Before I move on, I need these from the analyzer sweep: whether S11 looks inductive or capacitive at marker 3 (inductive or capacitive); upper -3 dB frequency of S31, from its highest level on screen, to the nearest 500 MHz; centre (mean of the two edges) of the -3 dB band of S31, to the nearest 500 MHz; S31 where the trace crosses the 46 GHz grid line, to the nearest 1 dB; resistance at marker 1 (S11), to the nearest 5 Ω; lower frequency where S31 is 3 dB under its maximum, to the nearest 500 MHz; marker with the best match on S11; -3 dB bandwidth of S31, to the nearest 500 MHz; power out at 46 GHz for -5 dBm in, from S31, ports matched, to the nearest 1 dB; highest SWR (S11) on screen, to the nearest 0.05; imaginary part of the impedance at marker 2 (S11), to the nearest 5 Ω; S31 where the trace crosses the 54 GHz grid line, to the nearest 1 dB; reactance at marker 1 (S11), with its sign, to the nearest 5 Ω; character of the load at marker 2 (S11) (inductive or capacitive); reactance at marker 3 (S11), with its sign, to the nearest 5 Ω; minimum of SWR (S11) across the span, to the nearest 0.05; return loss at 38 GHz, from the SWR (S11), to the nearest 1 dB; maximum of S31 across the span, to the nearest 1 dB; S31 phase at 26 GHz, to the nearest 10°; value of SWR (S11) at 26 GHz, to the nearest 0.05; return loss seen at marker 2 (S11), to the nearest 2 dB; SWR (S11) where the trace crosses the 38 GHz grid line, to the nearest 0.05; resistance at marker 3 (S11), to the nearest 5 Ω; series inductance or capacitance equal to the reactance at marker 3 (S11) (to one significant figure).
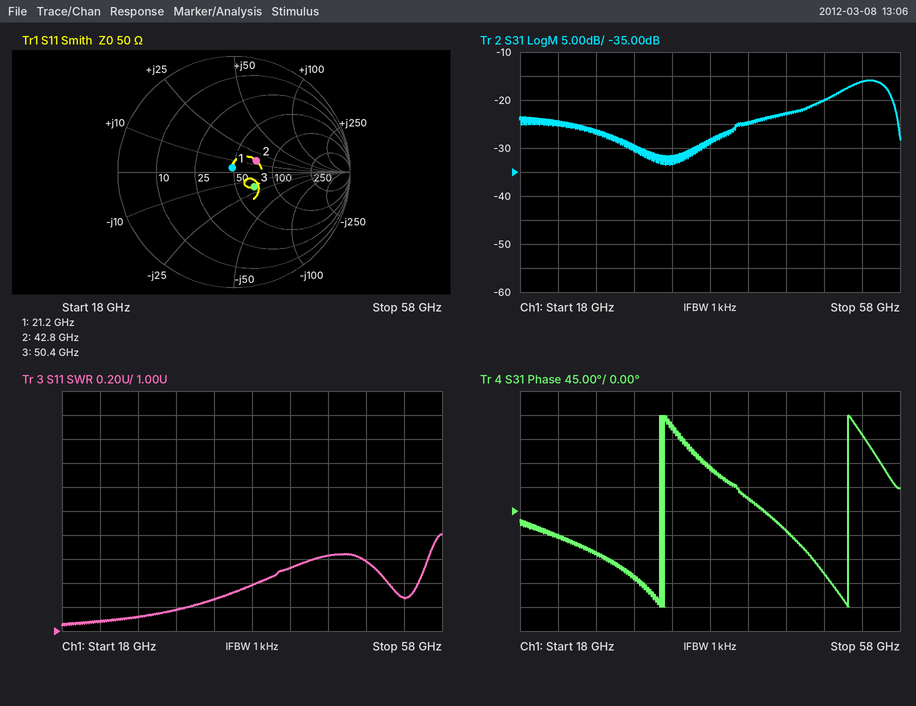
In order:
capacitive
57.0 GHz
54.0 GHz
-23 dB
50 Ω
51.0 GHz
marker 1
6.0 GHz
-28 dBm
1.80
+15 Ω
-16 dB
+5 Ω
inductive
-20 Ω
1.05
16 dB
-16 dB
-80°
1.10
14 dB
1.40
70 Ω
200 fF
